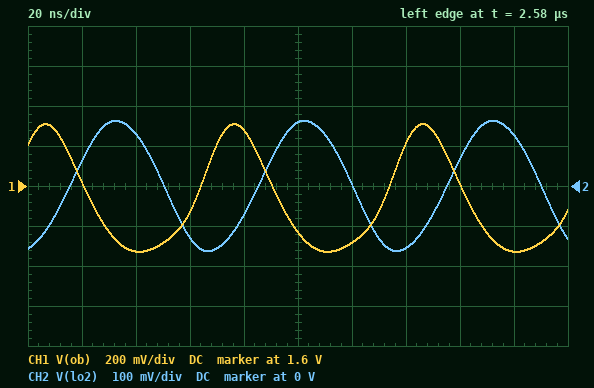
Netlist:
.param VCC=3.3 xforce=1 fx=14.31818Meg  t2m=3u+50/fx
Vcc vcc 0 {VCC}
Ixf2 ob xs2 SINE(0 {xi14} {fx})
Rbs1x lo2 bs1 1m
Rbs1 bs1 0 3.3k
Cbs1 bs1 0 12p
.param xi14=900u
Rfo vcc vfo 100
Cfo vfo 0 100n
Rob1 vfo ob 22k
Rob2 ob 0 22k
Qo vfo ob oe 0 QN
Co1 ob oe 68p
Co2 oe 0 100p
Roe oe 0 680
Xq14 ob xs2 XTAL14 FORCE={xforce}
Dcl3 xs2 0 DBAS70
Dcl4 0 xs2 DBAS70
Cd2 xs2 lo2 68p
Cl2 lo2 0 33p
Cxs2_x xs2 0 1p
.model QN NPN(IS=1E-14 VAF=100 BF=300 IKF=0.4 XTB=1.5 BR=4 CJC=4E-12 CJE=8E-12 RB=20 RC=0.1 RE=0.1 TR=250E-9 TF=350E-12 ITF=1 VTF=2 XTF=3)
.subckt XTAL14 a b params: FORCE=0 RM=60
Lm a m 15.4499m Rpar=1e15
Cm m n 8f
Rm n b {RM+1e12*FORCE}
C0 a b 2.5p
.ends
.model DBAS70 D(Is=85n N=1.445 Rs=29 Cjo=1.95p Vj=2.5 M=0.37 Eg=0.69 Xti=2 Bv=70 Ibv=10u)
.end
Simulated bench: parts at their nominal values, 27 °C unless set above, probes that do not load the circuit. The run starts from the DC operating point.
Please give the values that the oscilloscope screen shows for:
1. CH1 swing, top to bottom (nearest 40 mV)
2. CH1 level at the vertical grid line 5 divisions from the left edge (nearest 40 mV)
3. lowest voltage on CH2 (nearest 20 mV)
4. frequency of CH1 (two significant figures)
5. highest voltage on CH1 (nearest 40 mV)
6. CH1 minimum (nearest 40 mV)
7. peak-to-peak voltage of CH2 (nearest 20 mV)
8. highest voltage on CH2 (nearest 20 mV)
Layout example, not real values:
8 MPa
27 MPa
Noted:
640 mV
1.36 V
-160 mV
14 MHz
1.92 V
1.28 V
320 mV
160 mV
